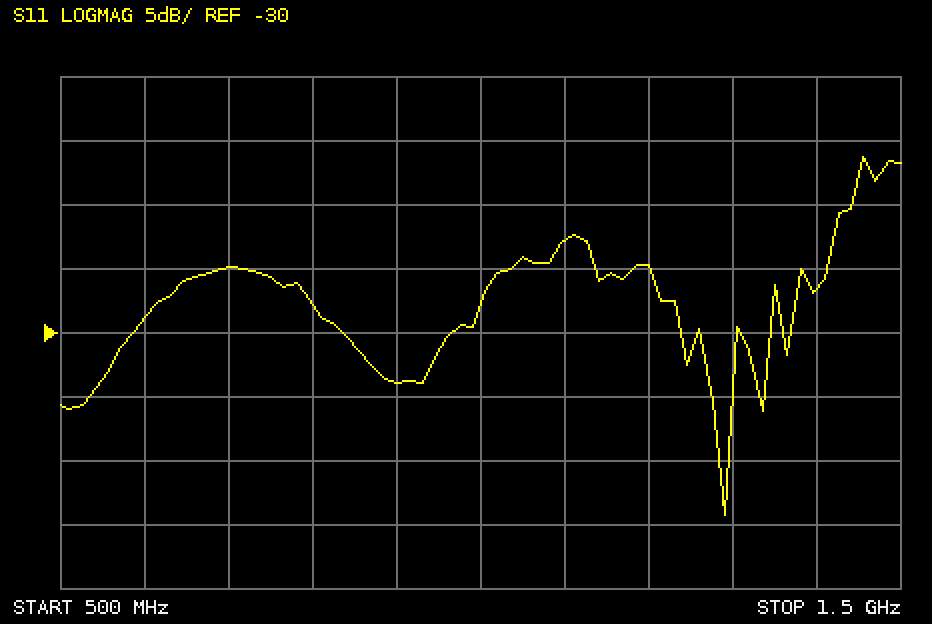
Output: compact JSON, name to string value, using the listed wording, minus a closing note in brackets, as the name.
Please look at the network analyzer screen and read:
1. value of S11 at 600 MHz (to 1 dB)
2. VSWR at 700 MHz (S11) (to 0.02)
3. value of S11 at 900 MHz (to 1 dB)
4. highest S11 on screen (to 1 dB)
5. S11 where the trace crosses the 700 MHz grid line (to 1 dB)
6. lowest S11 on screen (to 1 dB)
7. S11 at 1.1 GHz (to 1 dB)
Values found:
{"value of S11 at 600 MHz": "-29 dB", "VSWR at 700 MHz (S11)": "1.12", "value of S11 at 900 MHz": "-34 dB", "highest S11 on screen": "-16 dB", "S11 where the trace crosses the 700 MHz grid line": "-25 dB", "lowest S11 on screen": "-44 dB", "S11 at 1.1 GHz": "-23 dB"}
